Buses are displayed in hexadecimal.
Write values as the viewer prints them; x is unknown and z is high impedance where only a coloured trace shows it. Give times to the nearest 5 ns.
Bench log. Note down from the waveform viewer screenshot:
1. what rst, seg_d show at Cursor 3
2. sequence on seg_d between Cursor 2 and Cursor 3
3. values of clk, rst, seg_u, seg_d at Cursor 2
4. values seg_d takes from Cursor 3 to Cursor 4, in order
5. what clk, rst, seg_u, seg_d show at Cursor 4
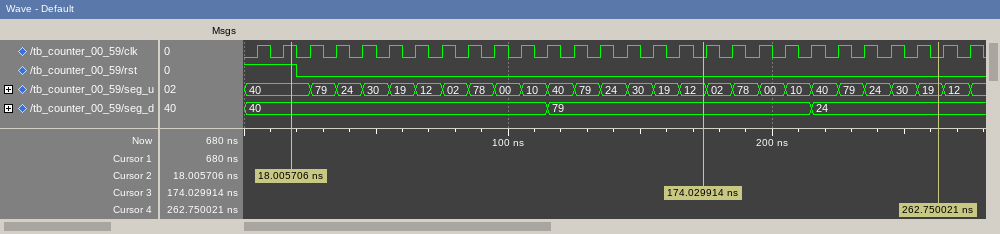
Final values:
rst=0, seg_d=79
40, 79
clk=1, rst=1, seg_u=40, seg_d=40
79, 24
clk=0, rst=0, seg_u=19, seg_d=24
